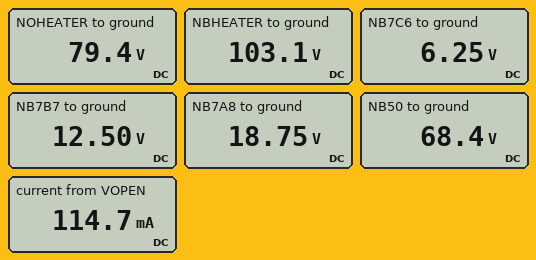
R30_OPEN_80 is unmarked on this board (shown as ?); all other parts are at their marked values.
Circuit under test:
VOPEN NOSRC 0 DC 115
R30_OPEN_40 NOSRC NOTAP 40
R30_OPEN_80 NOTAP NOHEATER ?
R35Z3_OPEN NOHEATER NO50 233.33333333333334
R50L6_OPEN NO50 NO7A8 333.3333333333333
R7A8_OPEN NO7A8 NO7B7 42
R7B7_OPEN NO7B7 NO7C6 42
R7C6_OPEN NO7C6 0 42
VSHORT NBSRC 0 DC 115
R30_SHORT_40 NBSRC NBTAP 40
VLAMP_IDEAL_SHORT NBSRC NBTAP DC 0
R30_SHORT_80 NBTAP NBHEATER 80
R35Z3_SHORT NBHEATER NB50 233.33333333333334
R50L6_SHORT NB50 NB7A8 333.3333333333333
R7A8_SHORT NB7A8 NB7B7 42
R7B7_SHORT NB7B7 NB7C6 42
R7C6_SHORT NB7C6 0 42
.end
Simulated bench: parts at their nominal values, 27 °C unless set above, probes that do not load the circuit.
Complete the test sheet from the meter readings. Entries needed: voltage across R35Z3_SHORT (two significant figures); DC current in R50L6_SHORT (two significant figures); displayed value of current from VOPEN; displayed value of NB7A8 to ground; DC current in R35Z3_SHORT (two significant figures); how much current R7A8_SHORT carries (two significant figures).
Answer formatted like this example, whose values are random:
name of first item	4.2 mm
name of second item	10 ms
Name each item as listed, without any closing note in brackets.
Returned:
voltage across R35Z3_SHORT	35 V
DC current in R50L6_SHORT	150 mA
displayed value of current from VOPEN	114.7 mA
displayed value of NB7A8 to ground	18.75 V
DC current in R35Z3_SHORT	150 mA
how much current R7A8_SHORT carries	150 mA
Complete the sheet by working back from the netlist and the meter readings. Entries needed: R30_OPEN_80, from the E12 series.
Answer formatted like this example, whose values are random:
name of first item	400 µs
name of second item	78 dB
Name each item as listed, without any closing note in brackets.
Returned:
R30_OPEN_80, from the E12 series	270 Ω
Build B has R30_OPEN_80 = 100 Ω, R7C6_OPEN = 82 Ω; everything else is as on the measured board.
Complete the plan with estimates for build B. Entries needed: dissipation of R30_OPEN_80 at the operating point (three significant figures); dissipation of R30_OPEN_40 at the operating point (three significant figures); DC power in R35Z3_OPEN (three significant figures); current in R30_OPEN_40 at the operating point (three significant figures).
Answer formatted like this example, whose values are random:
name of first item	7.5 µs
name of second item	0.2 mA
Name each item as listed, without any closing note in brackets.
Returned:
dissipation of R30_OPEN_80 at the operating point	1.74 W
dissipation of R30_OPEN_40 at the operating point	695 mW
DC power in R35Z3_OPEN	4.05 W
current in R30_OPEN_40 at the operating point	132 mA
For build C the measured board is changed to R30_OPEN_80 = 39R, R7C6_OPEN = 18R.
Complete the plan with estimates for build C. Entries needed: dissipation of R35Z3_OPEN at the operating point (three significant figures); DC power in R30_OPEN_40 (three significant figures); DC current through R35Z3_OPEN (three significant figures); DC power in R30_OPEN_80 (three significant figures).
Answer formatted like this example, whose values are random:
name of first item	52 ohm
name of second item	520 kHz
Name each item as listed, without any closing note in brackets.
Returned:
dissipation of R35Z3_OPEN at the operating point	5.52 W
DC power in R30_OPEN_40	946 mW
DC current through R35Z3_OPEN	154 mA
DC power in R30_OPEN_80	923 mW
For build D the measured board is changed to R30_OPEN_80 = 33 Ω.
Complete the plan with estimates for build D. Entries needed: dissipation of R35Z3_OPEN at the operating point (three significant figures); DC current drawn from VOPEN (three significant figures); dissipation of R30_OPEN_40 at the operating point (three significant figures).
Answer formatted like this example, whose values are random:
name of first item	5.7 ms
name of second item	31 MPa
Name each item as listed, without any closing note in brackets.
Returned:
dissipation of R35Z3_OPEN at the operating point	5.26 W
DC current drawn from VOPEN	150 mA
dissipation of R30_OPEN_40 at the operating point	902 mW
